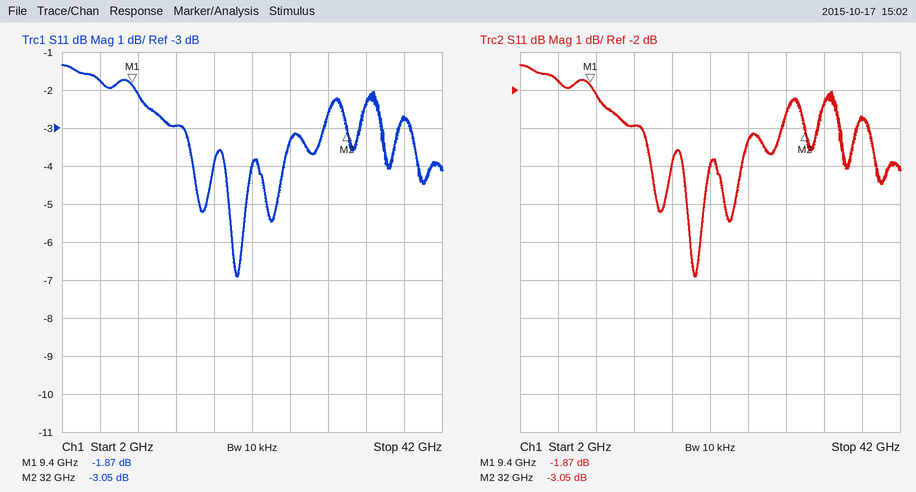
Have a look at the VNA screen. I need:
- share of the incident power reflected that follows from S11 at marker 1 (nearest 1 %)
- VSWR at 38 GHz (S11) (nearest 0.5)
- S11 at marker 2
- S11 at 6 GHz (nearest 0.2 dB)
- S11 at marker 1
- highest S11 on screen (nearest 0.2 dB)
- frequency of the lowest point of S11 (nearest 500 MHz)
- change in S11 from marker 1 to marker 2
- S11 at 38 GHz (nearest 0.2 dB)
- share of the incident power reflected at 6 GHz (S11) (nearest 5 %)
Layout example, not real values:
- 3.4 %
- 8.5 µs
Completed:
- 65 %
- 6.5
- -3.05 dB
- -1.8 dB
- -1.87 dB
- -1.4 dB
- 20.5 GHz
- -1.18 dB
- -2.8 dB
- 65 %
